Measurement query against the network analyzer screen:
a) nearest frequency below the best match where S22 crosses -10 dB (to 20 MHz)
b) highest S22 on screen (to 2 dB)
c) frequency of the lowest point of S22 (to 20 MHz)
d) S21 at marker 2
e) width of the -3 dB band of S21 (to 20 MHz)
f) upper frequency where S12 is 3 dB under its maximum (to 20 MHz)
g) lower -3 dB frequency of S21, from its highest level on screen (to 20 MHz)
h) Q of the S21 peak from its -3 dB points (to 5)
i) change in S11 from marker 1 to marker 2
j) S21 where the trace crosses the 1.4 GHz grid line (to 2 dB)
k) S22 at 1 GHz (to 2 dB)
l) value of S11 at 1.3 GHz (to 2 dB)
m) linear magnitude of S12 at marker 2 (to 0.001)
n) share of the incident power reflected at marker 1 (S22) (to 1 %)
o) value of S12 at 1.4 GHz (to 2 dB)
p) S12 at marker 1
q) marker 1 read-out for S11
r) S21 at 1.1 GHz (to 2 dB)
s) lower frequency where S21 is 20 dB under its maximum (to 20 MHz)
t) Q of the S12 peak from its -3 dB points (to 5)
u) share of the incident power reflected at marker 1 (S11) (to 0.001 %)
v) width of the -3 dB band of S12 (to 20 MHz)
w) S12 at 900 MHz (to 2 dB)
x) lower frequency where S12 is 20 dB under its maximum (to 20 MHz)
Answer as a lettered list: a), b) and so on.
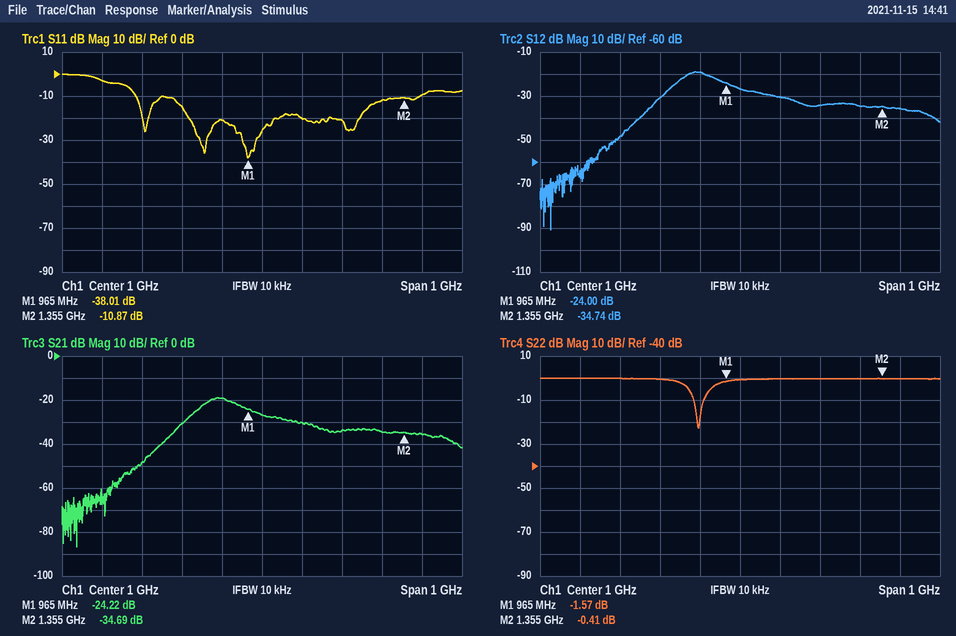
a) 880 MHz
b) 0 dB
c) 900 MHz
d) -34.69 dB
e) 80 MHz
f) 940 MHz
g) 860 MHz
h) 10
i) 27.14 dB
j) -36 dB
k) 0 dB
l) -12 dB
m) 0.018
n) 70 %
o) -36 dB
p) -24.00 dB
q) -38.01 dB
r) -30 dB
s) 760 MHz
t) 10
u) 0.016 %
v) 80 MHz
w) -20 dB
x) 760 MHz
